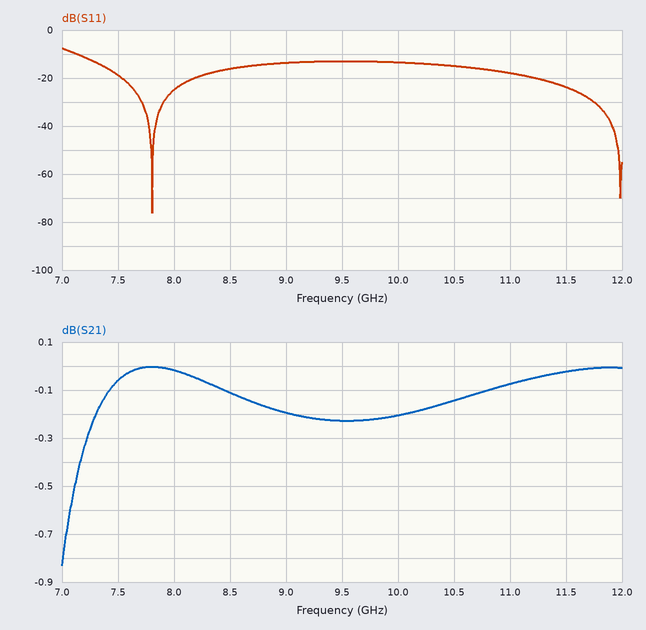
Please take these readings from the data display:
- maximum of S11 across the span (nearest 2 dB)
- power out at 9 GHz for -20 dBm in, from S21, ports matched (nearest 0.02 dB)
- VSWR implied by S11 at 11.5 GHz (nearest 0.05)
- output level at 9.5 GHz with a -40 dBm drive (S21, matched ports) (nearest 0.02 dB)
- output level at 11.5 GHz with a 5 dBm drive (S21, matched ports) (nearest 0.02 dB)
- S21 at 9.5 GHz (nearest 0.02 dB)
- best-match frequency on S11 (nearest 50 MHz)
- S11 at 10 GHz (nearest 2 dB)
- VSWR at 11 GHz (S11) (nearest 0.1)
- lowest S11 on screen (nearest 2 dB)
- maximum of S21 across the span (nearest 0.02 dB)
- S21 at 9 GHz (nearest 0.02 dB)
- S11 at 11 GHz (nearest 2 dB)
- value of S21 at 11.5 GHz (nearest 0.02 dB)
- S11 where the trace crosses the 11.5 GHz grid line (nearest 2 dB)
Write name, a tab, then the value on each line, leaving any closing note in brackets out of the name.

maximum of S11 across the span	-8 dB
power out at 9 GHz for -20 dBm in, from S21, ports matched	-20.20 dBm
VSWR implied by S11 at 11.5 GHz	1.15
output level at 9.5 GHz with a -40 dBm drive (S21, matched ports)	-40.22 dBm
output level at 11.5 GHz with a 5 dBm drive (S21, matched ports)	4.98 dBm
S21 at 9.5 GHz	-0.22 dB
best-match frequency on S11	7.80 GHz
S11 at 10 GHz	-14 dB
VSWR at 11 GHz (S11)	1.3
lowest S11 on screen	-76 dB
maximum of S21 across the span	0.00 dB
S21 at 9 GHz	-0.20 dB
S11 at 11 GHz	-18 dB
value of S21 at 11.5 GHz	-0.02 dB
S11 where the trace crosses the 11.5 GHz grid line	-24 dB
